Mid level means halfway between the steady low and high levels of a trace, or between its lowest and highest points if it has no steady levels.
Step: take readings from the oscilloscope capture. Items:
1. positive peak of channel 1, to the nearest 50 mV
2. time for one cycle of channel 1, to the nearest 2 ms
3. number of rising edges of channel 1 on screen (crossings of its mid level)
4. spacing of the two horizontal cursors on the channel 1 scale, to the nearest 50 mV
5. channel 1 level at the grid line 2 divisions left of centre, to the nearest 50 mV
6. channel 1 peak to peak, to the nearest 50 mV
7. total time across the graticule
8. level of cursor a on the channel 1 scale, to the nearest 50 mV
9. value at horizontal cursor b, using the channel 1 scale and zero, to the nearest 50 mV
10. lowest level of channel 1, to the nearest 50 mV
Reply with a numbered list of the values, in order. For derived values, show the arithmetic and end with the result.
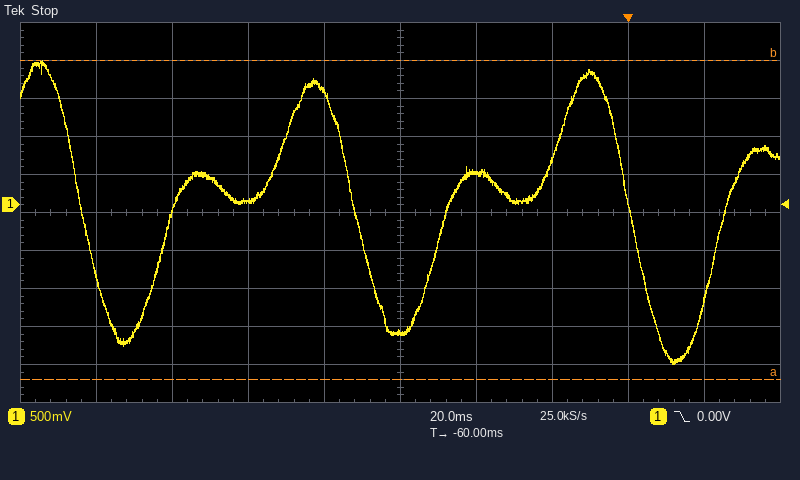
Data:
1. 1.90 V
2. 72 ms
3. 3
4. 4.20 V
5. 50 mV
6. 1.90 V − (-2.10 V) = 4.00 V
7. 200 ms
8. -2.30 V
9. 1.90 V
10. -2.10 V
